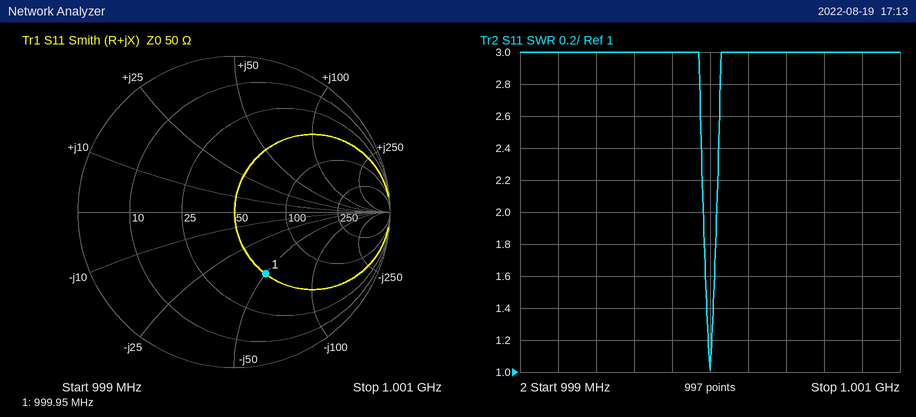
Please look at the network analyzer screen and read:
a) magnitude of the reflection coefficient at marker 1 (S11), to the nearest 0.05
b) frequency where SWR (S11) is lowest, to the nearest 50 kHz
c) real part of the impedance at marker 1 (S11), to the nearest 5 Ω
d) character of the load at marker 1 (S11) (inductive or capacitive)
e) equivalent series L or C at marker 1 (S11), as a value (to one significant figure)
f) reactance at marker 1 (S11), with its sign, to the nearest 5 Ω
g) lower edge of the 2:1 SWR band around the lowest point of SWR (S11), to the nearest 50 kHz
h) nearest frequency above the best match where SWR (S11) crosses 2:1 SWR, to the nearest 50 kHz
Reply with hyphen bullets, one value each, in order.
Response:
- 0.45
- 1.00000 GHz
- 50 Ω
- capacitive
- 3 pF
- -50 Ω
- 999.95 MHz
- 1.00005 GHz
